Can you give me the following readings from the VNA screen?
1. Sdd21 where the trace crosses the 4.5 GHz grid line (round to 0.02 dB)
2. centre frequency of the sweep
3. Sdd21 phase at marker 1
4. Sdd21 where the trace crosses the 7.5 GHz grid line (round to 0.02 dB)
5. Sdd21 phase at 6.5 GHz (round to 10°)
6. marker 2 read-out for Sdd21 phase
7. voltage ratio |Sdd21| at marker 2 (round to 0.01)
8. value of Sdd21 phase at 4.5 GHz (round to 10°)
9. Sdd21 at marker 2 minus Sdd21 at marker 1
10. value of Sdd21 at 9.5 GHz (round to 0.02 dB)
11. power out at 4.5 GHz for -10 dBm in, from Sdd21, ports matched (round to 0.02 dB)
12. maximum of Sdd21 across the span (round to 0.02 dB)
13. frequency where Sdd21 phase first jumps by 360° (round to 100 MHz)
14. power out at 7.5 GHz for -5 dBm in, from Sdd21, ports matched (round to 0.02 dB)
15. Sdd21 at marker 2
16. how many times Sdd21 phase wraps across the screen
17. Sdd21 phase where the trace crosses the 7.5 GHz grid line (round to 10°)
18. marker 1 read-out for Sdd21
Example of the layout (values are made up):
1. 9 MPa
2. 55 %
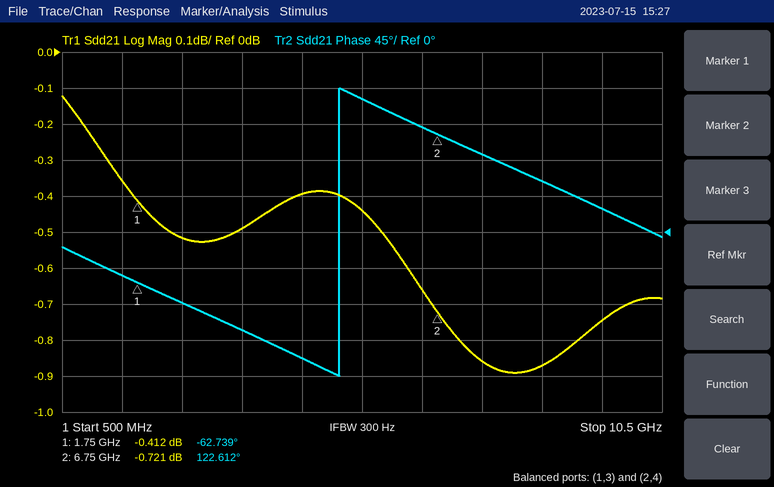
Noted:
1. -0.40 dB
2. 5.5 GHz
3. -62.739°
4. -0.86 dB
5. 130°
6. 122.612°
7. 0.92
8. -160°
9. -0.309 dB
10. -0.74 dB
11. -10.40 dBm
12. -0.12 dB
13. 5.1 GHz
14. -5.86 dBm
15. -0.721 dB
16. 1
17. 100°
18. -0.412 dB
